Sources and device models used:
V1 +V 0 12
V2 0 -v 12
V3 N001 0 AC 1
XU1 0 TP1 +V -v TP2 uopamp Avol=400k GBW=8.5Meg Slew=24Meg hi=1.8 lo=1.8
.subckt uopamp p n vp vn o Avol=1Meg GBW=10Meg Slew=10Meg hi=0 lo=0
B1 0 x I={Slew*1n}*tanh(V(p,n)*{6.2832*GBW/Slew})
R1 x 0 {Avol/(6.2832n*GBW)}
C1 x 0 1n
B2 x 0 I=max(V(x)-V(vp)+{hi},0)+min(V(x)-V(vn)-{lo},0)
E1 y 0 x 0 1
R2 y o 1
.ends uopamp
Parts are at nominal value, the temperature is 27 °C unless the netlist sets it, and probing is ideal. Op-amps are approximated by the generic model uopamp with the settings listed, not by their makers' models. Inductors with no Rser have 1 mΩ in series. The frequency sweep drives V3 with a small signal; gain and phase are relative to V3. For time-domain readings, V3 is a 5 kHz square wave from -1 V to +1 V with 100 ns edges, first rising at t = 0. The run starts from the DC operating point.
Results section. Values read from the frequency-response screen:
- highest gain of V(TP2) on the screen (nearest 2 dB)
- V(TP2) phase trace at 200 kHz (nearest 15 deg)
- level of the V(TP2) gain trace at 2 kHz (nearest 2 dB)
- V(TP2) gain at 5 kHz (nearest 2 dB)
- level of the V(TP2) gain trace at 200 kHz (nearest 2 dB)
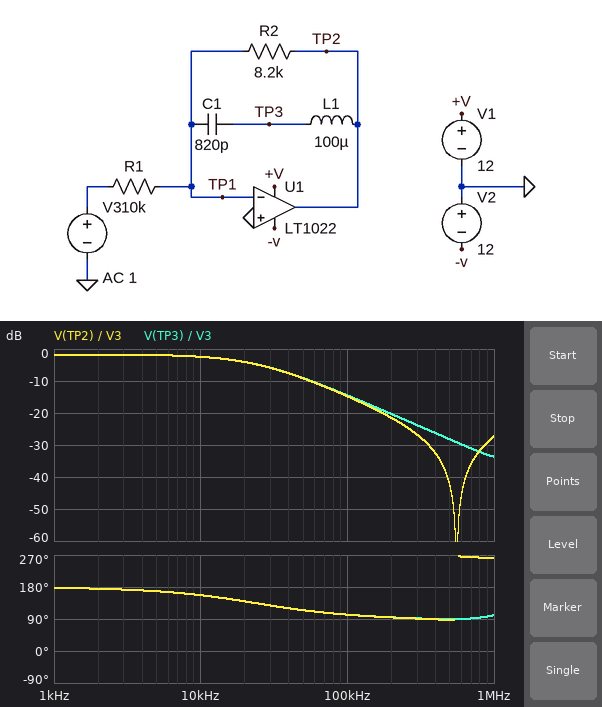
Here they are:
-2 dB
90 deg
-2 dB
-2 dB
-22 dB
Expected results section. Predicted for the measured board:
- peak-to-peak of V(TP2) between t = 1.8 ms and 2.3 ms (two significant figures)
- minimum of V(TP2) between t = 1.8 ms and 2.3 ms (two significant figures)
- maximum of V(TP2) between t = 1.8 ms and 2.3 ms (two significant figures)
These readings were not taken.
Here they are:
1.6 V
-820 mV
820 mV
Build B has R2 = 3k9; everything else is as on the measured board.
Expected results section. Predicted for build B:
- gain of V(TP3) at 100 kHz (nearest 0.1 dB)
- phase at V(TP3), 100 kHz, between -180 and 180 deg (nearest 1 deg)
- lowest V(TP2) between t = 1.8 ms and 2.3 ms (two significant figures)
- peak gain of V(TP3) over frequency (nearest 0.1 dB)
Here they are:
-15.2 dB
115 deg
-390 mV
-8.2 dB
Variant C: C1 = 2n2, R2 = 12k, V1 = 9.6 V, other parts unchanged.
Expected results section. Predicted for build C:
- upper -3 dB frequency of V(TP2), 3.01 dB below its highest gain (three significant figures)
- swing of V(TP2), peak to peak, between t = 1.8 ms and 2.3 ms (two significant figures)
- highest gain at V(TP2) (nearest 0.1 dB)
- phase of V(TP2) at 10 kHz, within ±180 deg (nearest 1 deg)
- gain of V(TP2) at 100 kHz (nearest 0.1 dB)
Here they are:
6.02 kHz
2.3 V
1.6 dB
121 deg
-23.6 dB
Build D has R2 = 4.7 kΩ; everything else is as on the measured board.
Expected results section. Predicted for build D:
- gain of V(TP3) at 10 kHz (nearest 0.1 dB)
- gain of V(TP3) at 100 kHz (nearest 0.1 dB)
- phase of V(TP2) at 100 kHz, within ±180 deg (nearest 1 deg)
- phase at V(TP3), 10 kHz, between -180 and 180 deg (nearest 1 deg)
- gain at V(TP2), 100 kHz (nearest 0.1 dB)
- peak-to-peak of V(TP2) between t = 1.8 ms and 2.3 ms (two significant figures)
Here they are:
-6.8 dB
-14.9 dB
111 deg
166 deg
-15.2 dB
940 mV
